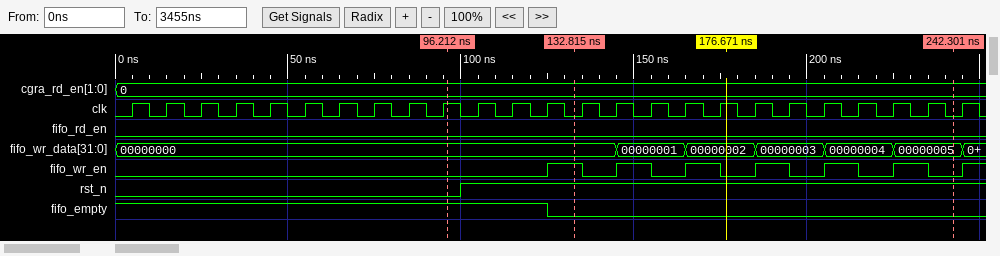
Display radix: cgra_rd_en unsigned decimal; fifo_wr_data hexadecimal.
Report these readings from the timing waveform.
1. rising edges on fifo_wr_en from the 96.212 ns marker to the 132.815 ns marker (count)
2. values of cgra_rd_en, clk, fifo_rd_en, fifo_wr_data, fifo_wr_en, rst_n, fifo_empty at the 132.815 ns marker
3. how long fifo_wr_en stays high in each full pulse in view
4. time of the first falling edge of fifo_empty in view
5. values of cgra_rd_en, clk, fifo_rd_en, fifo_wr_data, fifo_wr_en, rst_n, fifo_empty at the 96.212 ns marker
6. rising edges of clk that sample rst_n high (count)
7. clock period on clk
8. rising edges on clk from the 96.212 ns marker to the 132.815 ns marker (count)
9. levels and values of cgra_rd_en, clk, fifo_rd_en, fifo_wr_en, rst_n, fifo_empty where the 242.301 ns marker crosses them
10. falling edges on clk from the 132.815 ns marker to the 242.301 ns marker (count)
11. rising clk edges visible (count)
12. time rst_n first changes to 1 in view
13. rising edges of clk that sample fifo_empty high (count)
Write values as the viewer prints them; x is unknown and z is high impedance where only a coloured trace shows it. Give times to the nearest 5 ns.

1
cgra_rd_en=0, clk=0, fifo_rd_en=0, fifo_wr_data=00000000, fifo_wr_en=1, rst_n=1, fifo_empty=0
10 ns, 10 ns, 10 ns, 10 ns, 10 ns, 10 ns
125 ns
cgra_rd_en=0, clk=1, fifo_rd_en=0, fifo_wr_data=00000000, fifo_wr_en=0, rst_n=0, fifo_empty=1
15
10 ns
3
cgra_rd_en=0, clk=0, fifo_rd_en=0, fifo_wr_en=0, rst_n=1, fifo_empty=0
11
25
100 ns
13
